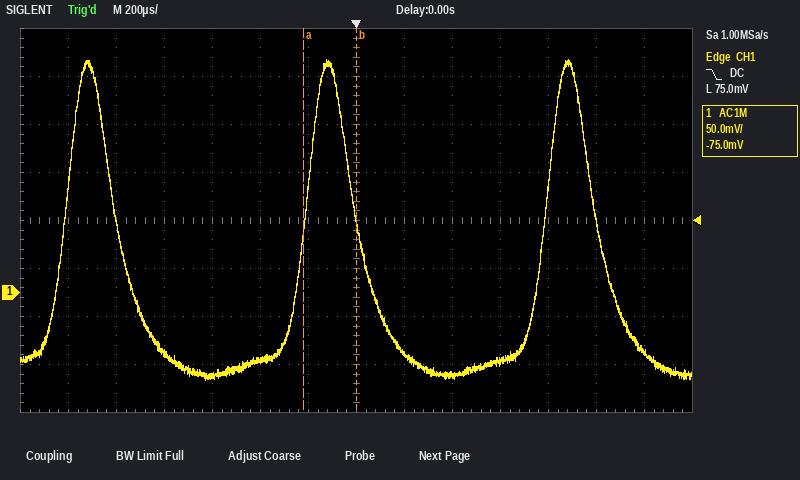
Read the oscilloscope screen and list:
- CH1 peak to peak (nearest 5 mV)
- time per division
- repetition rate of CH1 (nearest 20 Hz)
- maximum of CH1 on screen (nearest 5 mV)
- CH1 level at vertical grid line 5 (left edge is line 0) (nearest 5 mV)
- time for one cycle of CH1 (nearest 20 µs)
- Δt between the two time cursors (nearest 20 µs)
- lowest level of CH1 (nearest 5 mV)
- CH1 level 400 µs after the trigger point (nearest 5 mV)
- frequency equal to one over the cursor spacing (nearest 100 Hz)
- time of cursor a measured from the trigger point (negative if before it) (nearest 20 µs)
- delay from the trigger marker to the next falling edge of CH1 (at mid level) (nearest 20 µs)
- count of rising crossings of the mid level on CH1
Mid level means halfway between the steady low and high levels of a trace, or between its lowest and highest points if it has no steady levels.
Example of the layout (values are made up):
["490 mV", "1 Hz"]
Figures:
["335 mV", "200 µs", "1.00 kHz", "245 mV", "-70 mV", "1.00 ms", "220 µs", "-90 mV", "-85 mV", "4.5 kHz", "-220 µs", "1.00 ms", "3"]
